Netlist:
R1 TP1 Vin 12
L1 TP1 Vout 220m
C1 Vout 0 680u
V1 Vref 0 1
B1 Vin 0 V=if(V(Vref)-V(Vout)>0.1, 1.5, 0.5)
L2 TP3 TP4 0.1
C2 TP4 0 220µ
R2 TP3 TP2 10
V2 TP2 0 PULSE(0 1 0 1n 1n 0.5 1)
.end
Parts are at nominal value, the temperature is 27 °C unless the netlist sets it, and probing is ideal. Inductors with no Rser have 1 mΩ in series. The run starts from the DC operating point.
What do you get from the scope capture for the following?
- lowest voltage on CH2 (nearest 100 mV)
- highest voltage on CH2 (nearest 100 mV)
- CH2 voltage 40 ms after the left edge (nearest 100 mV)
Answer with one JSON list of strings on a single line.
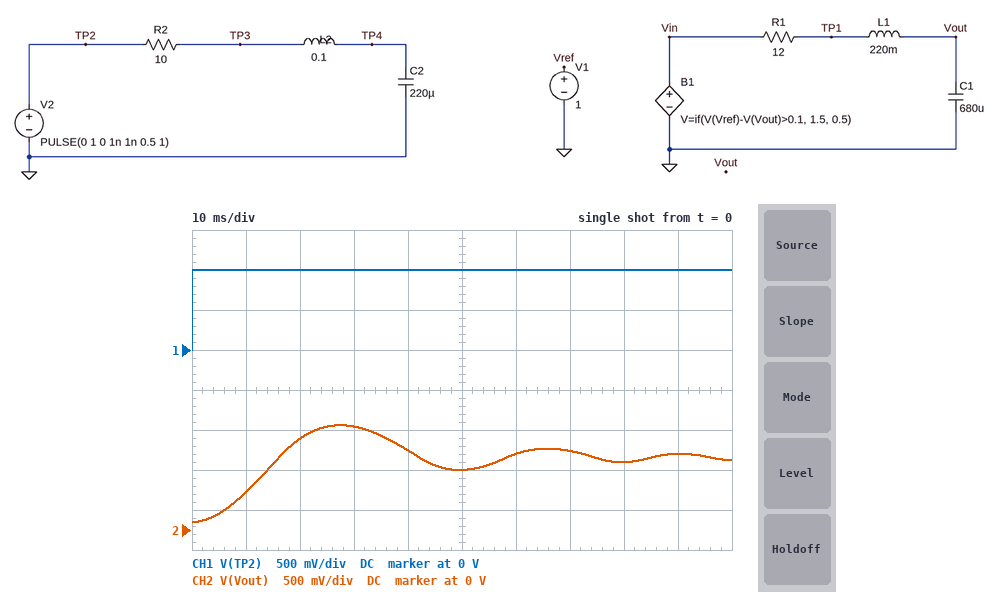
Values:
["100 mV", "1.3 V", "1.0 V"]
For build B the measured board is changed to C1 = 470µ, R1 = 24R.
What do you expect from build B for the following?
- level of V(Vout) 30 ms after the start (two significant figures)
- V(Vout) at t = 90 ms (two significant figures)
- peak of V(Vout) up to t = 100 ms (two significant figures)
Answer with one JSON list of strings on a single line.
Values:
["1.0 V", "900 mV", "1.1 V"]
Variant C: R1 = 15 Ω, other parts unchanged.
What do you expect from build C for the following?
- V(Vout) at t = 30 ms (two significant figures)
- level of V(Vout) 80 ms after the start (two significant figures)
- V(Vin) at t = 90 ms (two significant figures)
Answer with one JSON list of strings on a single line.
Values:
["1.2 V", "920 mV", "1.5 V"]
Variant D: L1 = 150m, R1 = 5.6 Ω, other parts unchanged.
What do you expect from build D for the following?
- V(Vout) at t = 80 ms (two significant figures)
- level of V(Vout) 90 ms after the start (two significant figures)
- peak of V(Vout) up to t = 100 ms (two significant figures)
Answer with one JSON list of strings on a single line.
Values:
["800 mV", "1.0 V", "1.5 V"]
